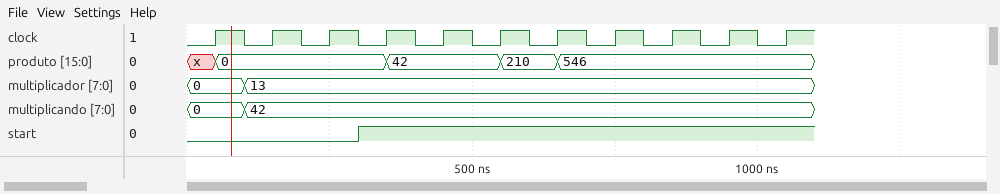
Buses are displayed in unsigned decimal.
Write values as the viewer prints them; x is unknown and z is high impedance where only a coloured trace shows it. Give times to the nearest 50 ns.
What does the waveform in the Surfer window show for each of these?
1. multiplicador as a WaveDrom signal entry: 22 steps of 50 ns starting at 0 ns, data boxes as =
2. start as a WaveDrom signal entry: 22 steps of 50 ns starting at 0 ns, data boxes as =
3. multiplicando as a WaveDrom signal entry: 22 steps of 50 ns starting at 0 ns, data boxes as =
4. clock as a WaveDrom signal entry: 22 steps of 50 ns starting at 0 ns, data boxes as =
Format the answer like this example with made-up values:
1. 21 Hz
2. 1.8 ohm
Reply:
1. {name: 'multiplicador', wave: '=.=...................', data: '0 13'}
2. {name: 'start', wave: '0.....1...............'}
3. {name: 'multiplicando', wave: '=.=...................', data: '0 42'}
4. {name: 'clock', wave: '0101010101010101010101'}
